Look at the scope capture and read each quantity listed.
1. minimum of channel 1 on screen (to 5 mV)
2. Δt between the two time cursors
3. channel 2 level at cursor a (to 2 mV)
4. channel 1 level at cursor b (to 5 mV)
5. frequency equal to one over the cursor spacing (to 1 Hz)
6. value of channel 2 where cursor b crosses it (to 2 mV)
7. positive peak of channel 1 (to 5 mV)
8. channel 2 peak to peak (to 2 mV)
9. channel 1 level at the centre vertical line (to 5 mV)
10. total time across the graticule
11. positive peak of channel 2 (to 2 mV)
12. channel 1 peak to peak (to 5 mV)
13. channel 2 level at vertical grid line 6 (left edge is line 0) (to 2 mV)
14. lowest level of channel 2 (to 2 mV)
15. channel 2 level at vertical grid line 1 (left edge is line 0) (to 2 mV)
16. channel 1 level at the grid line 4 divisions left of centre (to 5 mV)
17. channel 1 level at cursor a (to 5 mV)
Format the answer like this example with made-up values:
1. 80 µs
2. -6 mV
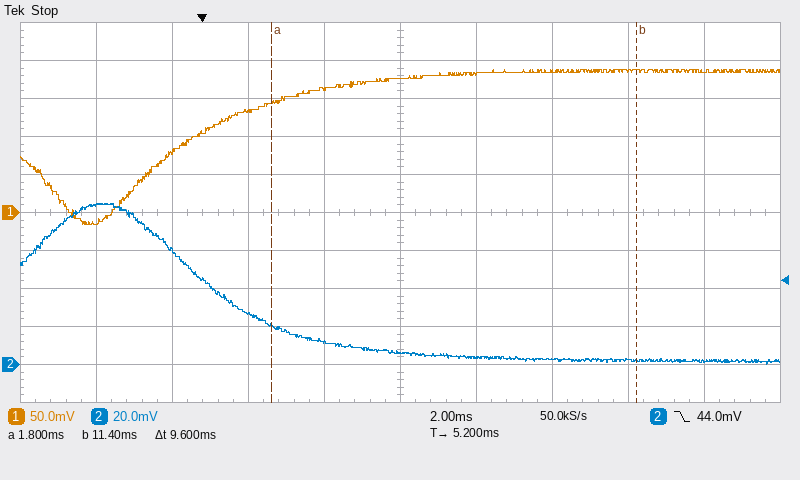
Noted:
1. -15 mV
2. 9.6 ms
3. 20 mV
4. 185 mV
5. 104 Hz
6. 2 mV
7. 190 mV
8. 84 mV
9. 175 mV
10. 20 ms
11. 84 mV
12. 205 mV
13. 4 mV
14. 0 mV
15. 84 mV
16. -10 mV
17. 145 mV
